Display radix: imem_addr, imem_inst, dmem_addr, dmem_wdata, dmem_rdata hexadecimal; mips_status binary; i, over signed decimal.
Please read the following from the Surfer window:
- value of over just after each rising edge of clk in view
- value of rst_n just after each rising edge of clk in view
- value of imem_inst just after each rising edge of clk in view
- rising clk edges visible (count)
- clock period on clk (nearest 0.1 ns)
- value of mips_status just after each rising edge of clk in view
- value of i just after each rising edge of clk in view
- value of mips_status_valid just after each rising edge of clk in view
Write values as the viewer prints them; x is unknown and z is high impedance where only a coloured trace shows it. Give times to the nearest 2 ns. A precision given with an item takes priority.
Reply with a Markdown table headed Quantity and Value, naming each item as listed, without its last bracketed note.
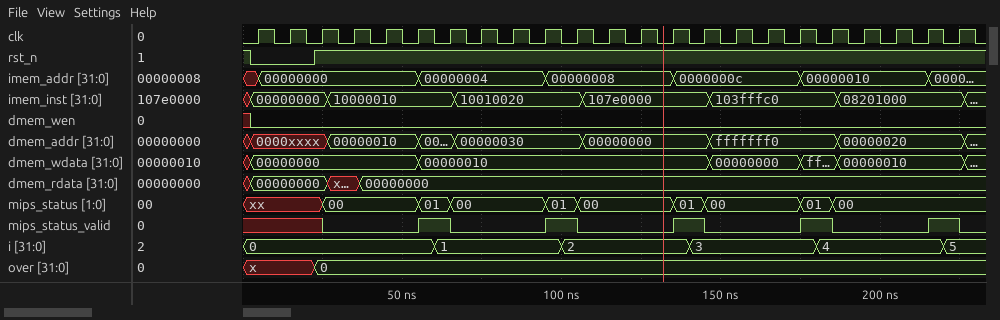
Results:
| Quantity | Value |
|---|---|
| value of over just after each rising edge of clk in view | x, x, 0, 0, 0, 0, 0, 0, 0, 0, 0, 0, 0, 0, 0, 0, 0, 0, 0, 0, 0, 0, 0 |
| value of rst_n just after each rising edge of clk in view | 0 0 1 1 1 1 1 1 1 1 1 1 1 1 1 1 1 1 1 1 1 1 1 |
| value of imem_inst just after each rising edge of clk in view | 00000000, 00000000, 00000000, 10000010, 10000010, 10000010, 10000010, 10010020, 10010020, 10010020, 10010020, 107e0000, 107e0000, 107e0000, 107e0000, 103fffc0, 103fffc0, 103fffc0, 103fffc0, 08201000, 08201000, 08201000, 08201000 |
| rising clk edges visible | 23 |
| clock period on clk | 10 ns |
| value of mips_status just after each rising edge of clk in view | xx, xx, 00, 00, 00, 01, 00, 00, 00, 01, 00, 00, 00, 01, 00, 00, 00, 01, 00, 00, 00, 00, 00 |
| value of i just after each rising edge of clk in view | 0, 0, 0, 0, 0, 0, 1, 1, 1, 1, 2, 2, 2, 2, 3, 3, 3, 3, 4, 4, 4, 4, 5 |
| value of mips_status_valid just after each rising edge of clk in view | x x 0 0 0 1 0 0 0 1 0 0 0 1 0 0 0 1 0 0 0 1 0 |
